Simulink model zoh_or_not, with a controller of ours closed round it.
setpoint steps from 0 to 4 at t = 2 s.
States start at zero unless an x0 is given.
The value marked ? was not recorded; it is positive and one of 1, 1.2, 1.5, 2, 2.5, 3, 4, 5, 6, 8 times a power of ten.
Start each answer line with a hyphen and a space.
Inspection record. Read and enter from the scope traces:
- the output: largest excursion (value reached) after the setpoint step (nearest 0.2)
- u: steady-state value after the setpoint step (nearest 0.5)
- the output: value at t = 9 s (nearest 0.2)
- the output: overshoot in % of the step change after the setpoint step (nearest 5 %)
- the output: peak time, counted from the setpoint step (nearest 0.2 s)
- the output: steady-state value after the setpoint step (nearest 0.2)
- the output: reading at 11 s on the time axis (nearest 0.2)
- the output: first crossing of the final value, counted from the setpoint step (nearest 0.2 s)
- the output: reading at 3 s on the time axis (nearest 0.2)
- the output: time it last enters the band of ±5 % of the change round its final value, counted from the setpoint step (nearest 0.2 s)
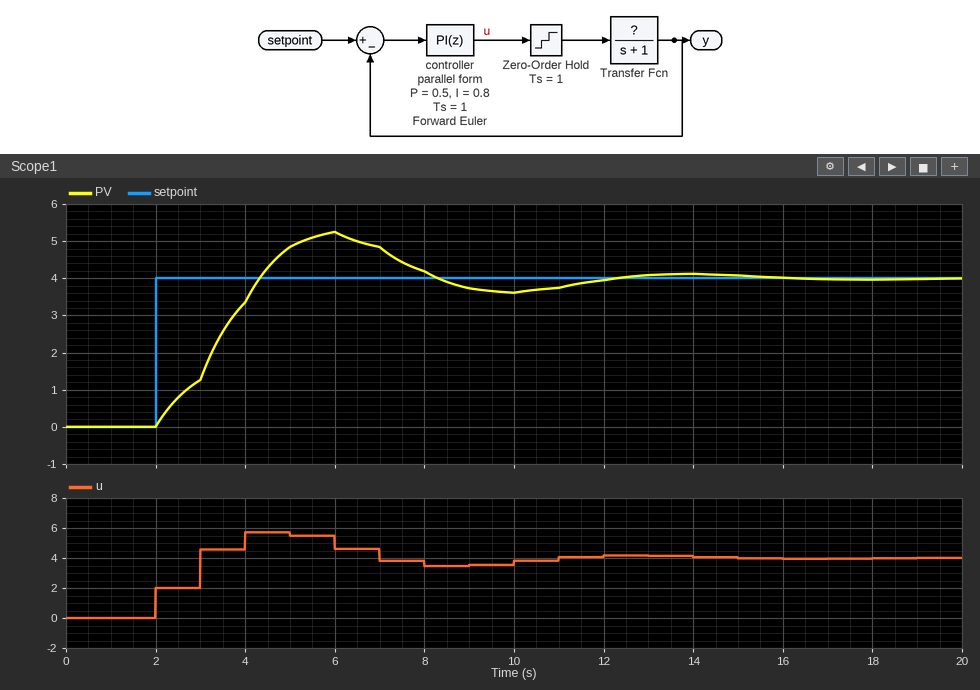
- 5.2
- 4.0
- 3.8
- 30 %
- 4.0 s
- 4.0
- 3.8
- 2.4 s
- 1.2
- 9.2 s
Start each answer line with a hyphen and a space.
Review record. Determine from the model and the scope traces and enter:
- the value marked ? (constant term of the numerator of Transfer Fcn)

- 1
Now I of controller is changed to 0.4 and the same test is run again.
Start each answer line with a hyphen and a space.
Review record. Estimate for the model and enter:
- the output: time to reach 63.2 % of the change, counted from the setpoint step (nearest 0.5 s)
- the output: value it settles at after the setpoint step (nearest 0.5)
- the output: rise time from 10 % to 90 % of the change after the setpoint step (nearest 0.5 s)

- 2.0 s
- 4.0
- 4.0 s
